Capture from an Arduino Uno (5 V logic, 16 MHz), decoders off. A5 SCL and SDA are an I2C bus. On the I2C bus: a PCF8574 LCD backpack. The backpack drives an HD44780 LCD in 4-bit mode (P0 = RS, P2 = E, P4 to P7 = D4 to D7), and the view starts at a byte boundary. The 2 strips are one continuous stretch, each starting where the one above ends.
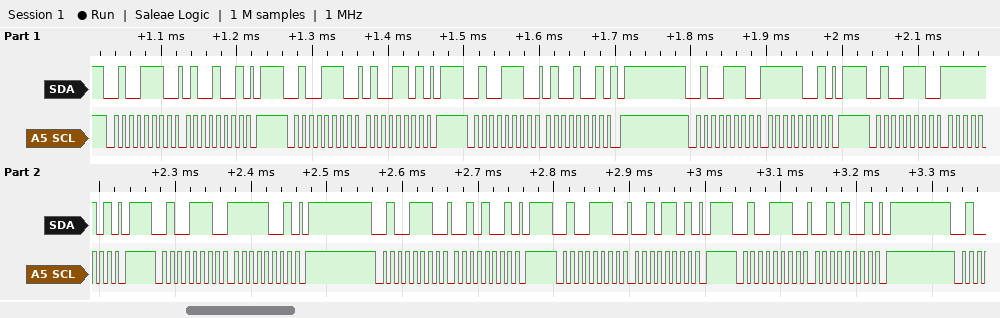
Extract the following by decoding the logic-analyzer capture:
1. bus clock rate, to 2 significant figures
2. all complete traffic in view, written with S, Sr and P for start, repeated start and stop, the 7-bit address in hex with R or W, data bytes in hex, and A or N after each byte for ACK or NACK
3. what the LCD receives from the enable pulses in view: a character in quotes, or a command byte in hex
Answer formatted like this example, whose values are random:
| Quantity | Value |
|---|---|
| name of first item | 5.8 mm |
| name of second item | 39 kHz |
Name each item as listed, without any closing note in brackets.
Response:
| Quantity | Value |
|---|---|
| bus clock rate, to 2 significant figures | 100 kHz |
| all complete traffic in view, written with S, Sr and P for start, repeated start and stop, the 7-bit address in hex with R or W, data bytes in hex, and A or N after each byte for ACK or NACK | S 27W A 49 A P S 27W A 4D A P S 27W A 49 A P S 27W A F9 A P S 27W A FD A P S 27W A F9 A P S 27W A 29 A P S 27W A 2D A P S 27W A 29 A P |
| what the LCD receives from the enable pulses in view: a character in quotes, or a command byte in hex | 'O' |
